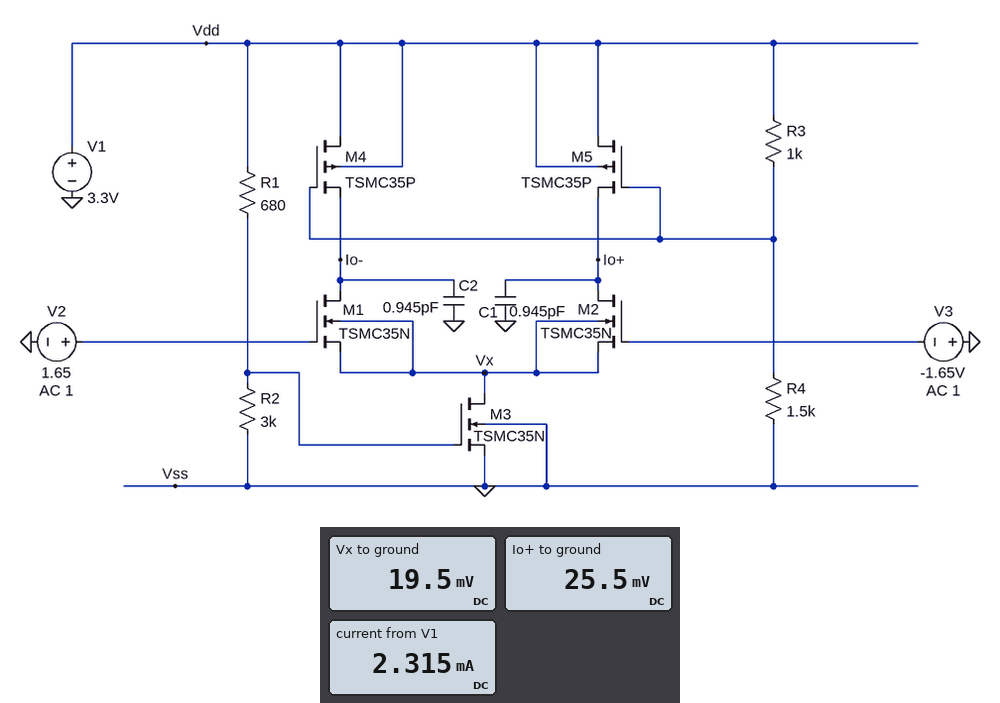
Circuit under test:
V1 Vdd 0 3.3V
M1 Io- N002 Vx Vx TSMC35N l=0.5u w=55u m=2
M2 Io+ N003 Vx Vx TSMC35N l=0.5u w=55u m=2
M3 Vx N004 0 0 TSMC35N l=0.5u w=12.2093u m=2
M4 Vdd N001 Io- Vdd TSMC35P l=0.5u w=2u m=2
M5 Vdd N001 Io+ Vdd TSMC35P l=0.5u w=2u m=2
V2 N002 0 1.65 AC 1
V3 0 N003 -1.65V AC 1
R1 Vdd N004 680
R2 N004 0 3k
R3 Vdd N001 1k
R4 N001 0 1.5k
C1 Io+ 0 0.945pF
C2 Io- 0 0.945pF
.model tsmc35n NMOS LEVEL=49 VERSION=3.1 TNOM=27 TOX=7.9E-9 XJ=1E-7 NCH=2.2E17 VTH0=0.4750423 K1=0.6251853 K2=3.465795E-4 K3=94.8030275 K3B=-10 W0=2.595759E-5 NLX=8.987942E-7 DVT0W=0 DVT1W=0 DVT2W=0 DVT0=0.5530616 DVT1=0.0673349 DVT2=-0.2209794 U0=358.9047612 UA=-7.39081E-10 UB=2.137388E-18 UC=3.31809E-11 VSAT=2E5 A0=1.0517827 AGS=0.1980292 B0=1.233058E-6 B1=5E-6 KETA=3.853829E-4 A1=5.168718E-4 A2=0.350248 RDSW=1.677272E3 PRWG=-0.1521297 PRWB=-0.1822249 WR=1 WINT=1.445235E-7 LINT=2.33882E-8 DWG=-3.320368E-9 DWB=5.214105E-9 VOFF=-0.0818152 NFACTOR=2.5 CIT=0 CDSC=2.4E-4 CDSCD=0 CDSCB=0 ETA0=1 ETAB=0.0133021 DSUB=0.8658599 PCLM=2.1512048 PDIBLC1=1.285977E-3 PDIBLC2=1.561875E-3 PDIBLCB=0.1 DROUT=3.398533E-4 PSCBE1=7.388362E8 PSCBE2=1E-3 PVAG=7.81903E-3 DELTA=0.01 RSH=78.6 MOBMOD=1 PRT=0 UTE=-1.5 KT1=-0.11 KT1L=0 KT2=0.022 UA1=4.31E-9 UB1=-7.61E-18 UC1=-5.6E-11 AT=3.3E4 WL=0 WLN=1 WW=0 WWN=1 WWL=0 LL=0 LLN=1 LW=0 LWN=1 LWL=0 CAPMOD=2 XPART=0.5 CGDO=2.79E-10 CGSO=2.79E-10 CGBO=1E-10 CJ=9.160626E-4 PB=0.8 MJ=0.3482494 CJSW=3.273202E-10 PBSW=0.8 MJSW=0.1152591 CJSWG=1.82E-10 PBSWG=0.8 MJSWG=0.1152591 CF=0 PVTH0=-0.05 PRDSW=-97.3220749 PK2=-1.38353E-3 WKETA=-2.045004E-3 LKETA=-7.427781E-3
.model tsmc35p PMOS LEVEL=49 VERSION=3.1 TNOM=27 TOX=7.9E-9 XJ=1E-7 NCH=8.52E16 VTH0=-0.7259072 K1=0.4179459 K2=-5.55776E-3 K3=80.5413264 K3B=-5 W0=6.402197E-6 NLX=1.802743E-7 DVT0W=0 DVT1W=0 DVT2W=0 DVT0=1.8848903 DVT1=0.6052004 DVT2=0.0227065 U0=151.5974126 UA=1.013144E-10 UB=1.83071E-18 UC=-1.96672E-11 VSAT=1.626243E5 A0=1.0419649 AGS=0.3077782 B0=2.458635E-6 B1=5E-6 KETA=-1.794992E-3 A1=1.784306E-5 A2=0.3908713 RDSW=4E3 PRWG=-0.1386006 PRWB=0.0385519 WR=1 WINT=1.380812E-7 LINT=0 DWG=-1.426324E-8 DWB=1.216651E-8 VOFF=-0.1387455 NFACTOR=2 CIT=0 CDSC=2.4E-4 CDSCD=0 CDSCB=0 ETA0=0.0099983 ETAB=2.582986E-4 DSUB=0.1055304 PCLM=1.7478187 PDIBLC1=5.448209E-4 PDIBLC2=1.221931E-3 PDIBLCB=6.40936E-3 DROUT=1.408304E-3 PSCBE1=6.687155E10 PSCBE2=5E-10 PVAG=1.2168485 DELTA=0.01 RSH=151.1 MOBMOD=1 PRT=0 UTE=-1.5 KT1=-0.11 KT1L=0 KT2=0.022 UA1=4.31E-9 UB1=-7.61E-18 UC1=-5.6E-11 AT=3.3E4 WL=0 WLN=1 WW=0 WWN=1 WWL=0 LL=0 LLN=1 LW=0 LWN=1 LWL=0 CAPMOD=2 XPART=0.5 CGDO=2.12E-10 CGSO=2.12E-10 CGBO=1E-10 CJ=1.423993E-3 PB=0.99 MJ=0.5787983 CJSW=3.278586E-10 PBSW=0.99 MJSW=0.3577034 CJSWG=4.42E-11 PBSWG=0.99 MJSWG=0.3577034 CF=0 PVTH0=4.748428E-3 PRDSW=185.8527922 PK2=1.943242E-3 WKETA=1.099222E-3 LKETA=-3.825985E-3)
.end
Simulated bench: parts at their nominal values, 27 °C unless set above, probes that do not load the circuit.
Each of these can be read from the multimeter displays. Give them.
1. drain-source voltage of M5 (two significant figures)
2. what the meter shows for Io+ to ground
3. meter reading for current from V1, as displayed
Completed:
3.3 V
25.5 mV
2.315 mA
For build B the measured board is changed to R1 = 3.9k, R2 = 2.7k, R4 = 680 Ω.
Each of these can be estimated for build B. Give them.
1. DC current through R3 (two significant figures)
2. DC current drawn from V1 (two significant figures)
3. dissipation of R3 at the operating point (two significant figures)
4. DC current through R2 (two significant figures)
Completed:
2.0 mA
2.8 mA
3.9 mW
500 µA
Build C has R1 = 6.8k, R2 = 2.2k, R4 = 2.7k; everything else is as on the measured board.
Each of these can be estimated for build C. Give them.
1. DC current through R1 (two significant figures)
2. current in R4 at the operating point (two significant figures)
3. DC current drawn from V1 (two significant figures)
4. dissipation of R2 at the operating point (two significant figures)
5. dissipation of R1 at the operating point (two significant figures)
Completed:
370 µA
890 µA
1.3 mA
300 µW
910 µW
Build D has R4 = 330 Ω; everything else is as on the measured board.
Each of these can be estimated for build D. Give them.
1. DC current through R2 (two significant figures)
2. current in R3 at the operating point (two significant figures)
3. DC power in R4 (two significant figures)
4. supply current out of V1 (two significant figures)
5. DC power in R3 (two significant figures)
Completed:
900 µA
2.5 mA
2.0 mW
4.0 mA
6.2 mW
